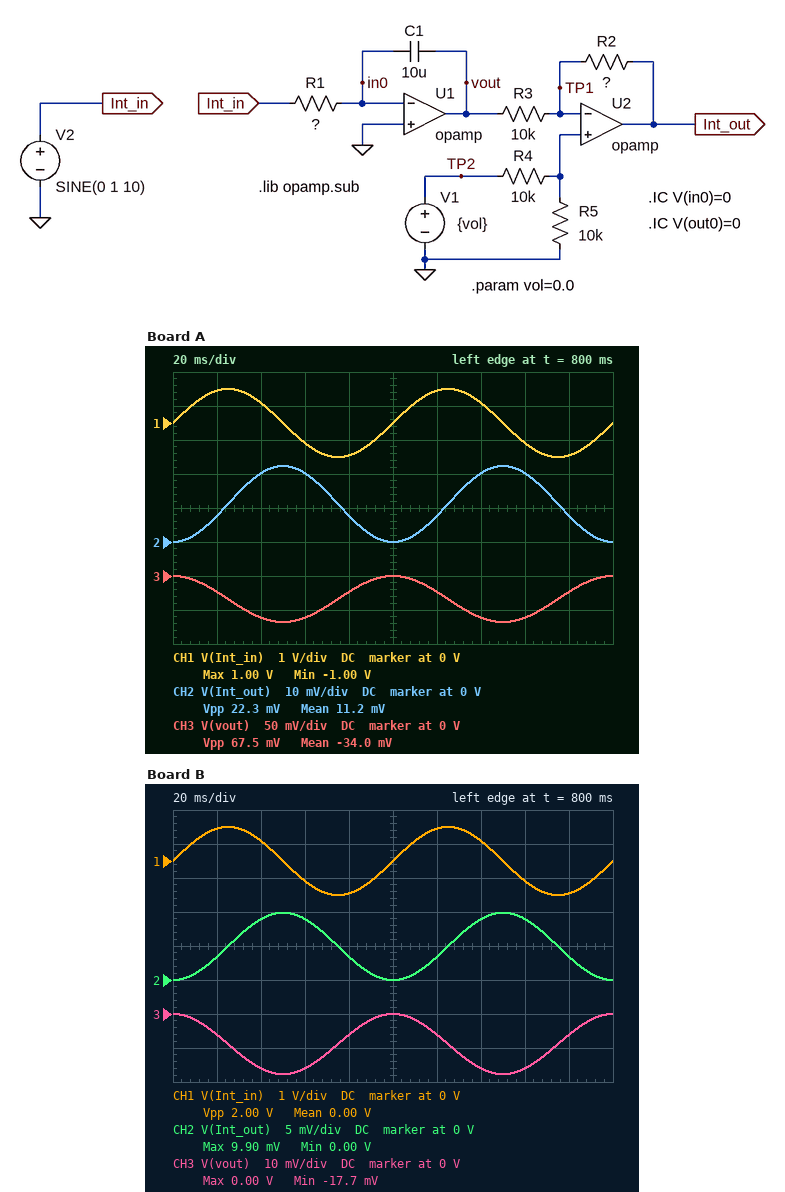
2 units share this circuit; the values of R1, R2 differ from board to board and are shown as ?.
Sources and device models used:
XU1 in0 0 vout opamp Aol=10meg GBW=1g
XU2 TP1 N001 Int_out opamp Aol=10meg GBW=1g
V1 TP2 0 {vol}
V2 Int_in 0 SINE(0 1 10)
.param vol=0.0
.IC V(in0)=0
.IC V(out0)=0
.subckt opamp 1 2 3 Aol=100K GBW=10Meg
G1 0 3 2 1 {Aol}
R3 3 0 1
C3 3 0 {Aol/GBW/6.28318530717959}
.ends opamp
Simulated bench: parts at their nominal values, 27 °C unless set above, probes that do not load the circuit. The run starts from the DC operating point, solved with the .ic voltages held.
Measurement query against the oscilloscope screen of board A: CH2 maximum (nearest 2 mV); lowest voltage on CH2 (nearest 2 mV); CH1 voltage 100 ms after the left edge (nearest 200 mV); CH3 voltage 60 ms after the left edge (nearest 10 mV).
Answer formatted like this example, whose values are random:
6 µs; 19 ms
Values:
22 mV; 0 V; 0 V; -60 mV
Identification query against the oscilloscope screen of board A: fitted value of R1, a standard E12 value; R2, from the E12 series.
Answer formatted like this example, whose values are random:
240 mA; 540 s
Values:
47 kΩ; 3.3 kΩ
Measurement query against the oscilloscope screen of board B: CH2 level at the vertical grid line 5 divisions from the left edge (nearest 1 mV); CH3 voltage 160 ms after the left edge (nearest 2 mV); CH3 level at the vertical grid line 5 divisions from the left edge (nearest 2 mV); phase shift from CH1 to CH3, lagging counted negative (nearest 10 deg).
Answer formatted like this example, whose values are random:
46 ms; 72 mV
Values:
0 V; -16 mV; 0 V; 90 deg
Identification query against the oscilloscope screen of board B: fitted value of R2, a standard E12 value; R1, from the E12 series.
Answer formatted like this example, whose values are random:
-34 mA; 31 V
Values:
5.6 kΩ; 180 kΩ
